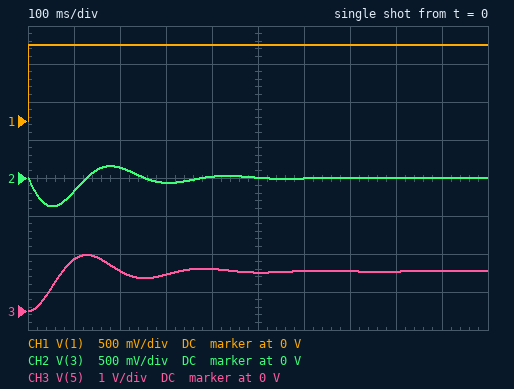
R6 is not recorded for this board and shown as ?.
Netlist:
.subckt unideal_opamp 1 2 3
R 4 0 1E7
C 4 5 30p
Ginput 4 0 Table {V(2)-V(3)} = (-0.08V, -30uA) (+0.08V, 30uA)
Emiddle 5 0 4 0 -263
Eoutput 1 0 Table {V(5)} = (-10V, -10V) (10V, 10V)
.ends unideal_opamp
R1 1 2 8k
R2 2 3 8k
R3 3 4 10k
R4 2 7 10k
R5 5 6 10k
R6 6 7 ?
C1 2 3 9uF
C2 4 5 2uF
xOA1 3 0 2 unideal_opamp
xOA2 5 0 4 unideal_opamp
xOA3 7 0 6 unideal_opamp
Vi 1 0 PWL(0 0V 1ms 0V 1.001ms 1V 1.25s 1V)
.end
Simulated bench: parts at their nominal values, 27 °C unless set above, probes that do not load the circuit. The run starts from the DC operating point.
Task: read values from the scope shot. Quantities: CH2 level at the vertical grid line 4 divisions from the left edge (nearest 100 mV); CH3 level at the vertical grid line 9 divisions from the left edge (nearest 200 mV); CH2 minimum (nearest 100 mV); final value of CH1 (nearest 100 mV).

0 V
1.0 V
-400 mV
1.0 V
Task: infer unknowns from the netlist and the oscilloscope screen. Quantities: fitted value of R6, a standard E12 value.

12 kΩ
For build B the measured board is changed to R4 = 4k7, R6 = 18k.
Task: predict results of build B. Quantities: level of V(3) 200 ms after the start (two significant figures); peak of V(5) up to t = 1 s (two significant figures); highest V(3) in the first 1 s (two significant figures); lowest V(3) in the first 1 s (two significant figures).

-26 mV
530 mV
150 mV
-240 mV
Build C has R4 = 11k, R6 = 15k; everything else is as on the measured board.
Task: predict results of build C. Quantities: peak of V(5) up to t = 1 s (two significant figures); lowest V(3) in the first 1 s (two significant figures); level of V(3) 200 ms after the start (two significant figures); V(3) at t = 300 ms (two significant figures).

1.3 V
-360 mV
110 mV
-65 mV
